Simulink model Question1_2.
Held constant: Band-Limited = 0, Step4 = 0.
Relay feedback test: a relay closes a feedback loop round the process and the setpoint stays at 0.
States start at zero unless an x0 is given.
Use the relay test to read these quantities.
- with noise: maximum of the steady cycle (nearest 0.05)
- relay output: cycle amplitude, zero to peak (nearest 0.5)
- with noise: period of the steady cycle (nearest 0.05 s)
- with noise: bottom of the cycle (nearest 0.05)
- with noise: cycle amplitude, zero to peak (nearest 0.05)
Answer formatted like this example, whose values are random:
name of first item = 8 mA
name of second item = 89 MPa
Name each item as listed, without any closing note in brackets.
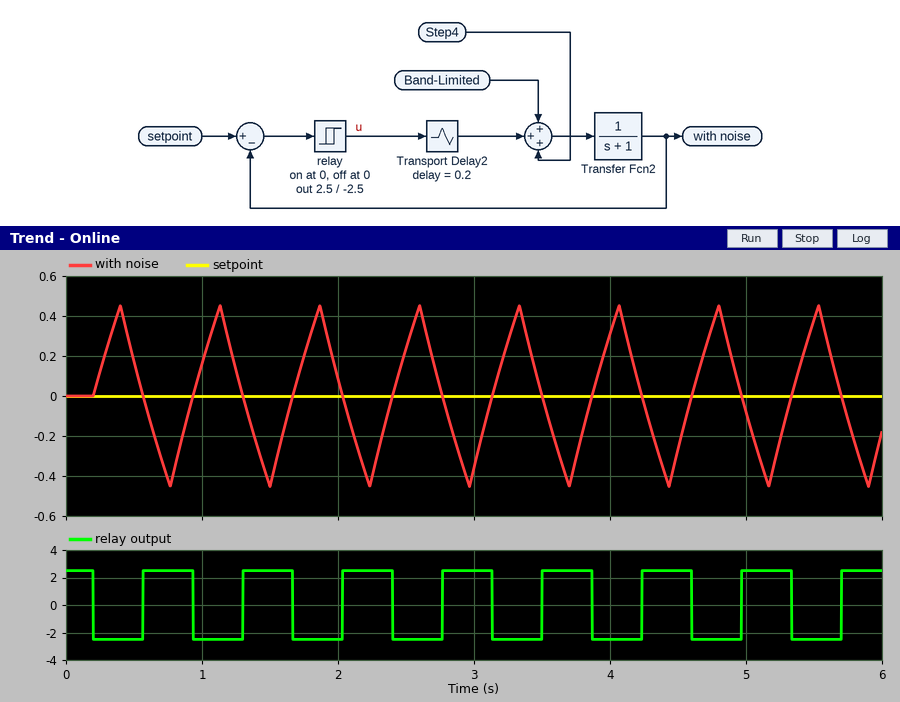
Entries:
with noise: maximum of the steady cycle = 0.45
relay output: cycle amplitude, zero to peak = 2.5
with noise: period of the steady cycle = 0.75 s
with noise: bottom of the cycle = -0.45
with noise: cycle amplitude, zero to peak = 0.45
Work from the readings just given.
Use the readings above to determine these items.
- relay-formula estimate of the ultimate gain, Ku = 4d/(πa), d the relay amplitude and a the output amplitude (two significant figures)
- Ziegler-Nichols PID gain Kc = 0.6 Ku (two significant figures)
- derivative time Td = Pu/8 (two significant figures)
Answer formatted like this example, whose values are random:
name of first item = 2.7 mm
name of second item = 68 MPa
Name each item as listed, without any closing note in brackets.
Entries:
relay-formula estimate of the ultimate gain, Ku = 4d/(πa), d the relay amplitude and a the output amplitude = 7.1
Ziegler-Nichols PID gain Kc = 0.6 Ku = 4.3
derivative time Td = Pu/8 = 0.094 s
